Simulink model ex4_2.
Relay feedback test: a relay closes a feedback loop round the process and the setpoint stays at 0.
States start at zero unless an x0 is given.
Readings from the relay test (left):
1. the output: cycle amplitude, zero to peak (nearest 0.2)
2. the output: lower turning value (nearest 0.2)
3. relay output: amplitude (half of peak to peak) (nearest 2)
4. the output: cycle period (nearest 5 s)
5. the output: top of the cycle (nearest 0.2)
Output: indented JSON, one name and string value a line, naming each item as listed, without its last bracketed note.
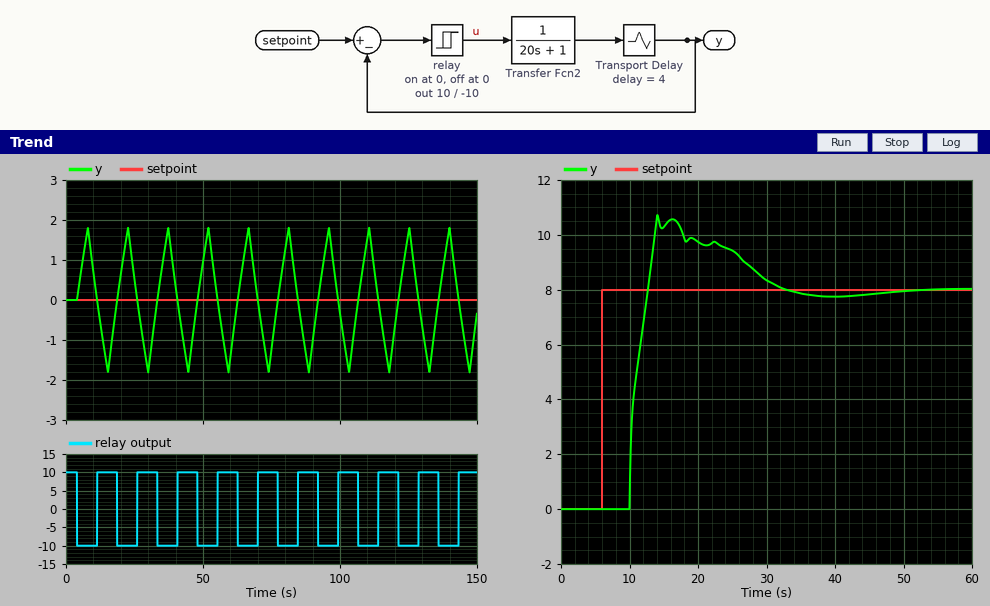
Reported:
{
  "the output: cycle amplitude, zero to peak": "1.8",
  "the output: lower turning value": "-1.8",
  "relay output: amplitude (half of peak to peak)": "10",
  "the output: cycle period": "15 s",
  "the output: top of the cycle": "1.8"
}
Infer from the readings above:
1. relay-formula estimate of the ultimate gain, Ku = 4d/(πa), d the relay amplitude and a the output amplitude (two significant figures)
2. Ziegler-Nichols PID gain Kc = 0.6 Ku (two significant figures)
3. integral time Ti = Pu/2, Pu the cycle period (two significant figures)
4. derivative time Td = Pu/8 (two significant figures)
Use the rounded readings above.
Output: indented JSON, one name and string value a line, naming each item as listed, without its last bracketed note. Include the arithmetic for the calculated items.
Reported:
{
  "relay-formula estimate of the ultimate gain, Ku = 4d/(πa), d the relay amplitude and a the output amplitude": "4 × 10 / (π × 1.8) = 7.1",
  "Ziegler-Nichols PID gain Kc = 0.6 Ku": "0.6 × 7.1 = 4.3",
  "integral time Ti = Pu/2, Pu the cycle period": "15 / 2 = 7.5 s",
  "derivative time Td = Pu/8": "15 / 8 = 1.9 s"
}
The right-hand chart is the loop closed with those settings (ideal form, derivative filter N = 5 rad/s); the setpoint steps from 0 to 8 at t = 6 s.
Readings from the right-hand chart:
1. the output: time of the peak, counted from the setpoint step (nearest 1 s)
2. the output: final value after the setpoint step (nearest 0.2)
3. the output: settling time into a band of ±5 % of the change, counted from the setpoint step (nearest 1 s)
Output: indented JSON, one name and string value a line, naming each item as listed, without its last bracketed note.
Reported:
{
  "the output: time of the peak, counted from the setpoint step": "8 s",
  "the output: final value after the setpoint step": "8.0",
  "the output: settling time into a band of ±5 % of the change, counted from the setpoint step": "24 s"
}
